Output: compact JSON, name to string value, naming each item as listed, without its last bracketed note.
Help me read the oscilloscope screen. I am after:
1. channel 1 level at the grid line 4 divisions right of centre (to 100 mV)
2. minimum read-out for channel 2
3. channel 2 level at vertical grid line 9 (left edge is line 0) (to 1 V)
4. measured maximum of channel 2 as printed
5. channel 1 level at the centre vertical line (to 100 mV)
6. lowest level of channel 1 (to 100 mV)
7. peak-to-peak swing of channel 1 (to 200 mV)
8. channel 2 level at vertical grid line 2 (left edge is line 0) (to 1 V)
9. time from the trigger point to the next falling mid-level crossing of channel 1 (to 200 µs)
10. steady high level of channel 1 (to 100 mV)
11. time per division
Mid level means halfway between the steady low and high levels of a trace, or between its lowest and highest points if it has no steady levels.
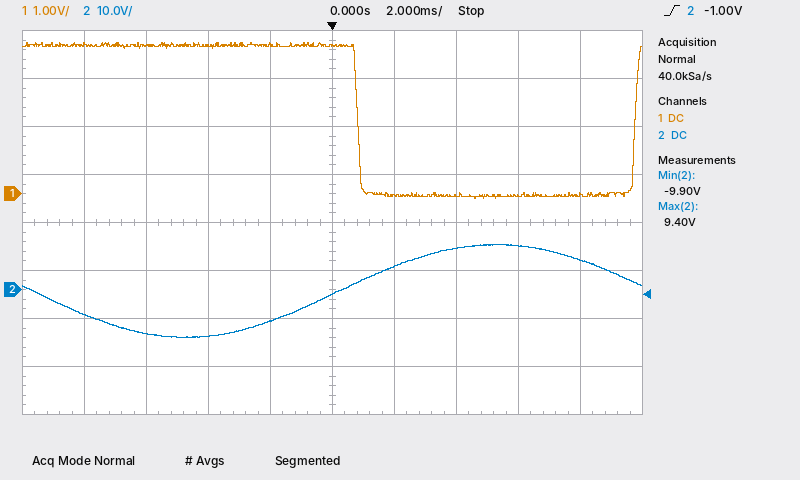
{"channel 1 level at the grid line 4 divisions right of centre": "0.0 V", "minimum read-out for channel 2": "-9.90 V", "channel 2 level at vertical grid line 9 (left edge is line 0)": "6 V", "measured maximum of channel 2 as printed": "9.40 V", "channel 1 level at the centre vertical line": "3.1 V", "lowest level of channel 1": "-100 mV", "peak-to-peak swing of channel 1": "3.2 V", "channel 2 level at vertical grid line 2 (left edge is line 0)": "-9 V", "time from the trigger point to the next falling mid-level crossing of channel 1": "800 µs", "steady high level of channel 1": "3.1 V", "time per division": "2 ms"}
